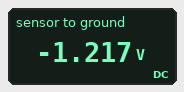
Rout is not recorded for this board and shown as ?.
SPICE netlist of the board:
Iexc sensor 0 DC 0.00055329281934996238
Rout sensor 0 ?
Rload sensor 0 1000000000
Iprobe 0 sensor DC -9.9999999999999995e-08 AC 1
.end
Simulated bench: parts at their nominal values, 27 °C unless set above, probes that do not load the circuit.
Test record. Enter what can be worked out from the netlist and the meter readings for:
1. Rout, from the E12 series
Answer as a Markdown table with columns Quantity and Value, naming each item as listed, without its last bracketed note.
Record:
| Quantity | Value |
|---|---|
| Rout, from the E12 series | 2.2 kΩ |
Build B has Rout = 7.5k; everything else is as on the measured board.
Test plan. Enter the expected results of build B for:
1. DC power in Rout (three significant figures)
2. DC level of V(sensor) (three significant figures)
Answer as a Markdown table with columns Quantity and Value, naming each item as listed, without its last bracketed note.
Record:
| Quantity | Value |
|---|---|
| DC power in Rout | 2.30 mW |
| DC level of V(sensor) | -4.15 V |
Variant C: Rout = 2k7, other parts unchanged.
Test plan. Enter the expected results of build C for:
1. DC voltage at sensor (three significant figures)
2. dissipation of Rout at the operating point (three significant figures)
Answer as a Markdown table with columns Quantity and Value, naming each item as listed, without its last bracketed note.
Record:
| Quantity | Value |
|---|---|
| DC voltage at sensor | -1.49 V |
| dissipation of Rout at the operating point | 827 µW |
